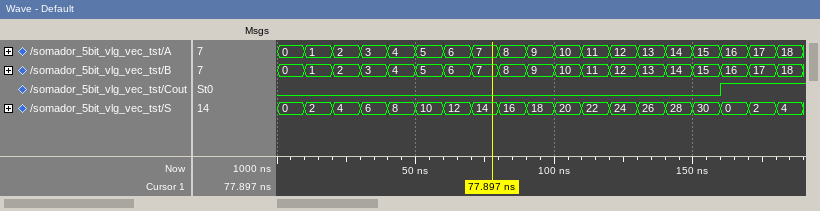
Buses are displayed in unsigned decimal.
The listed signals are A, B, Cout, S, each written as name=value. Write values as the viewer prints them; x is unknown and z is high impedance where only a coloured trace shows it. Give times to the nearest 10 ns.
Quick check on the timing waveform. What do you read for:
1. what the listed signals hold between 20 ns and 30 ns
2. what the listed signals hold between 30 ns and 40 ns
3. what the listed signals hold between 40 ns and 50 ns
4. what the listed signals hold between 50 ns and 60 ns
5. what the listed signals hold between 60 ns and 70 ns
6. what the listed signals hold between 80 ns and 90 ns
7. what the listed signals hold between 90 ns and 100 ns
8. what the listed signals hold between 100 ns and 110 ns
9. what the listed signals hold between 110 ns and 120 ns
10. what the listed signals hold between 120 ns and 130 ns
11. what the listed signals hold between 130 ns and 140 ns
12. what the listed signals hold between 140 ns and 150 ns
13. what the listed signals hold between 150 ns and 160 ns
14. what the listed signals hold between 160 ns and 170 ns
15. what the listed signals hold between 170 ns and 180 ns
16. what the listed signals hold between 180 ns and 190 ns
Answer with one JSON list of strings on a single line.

["A=2, B=2, Cout=0, S=4", "A=3, B=3, Cout=0, S=6", "A=4, B=4, Cout=0, S=8", "A=5, B=5, Cout=0, S=10", "A=6, B=6, Cout=0, S=12", "A=8, B=8, Cout=0, S=16", "A=9, B=9, Cout=0, S=18", "A=10, B=10, Cout=0, S=20", "A=11, B=11, Cout=0, S=22", "A=12, B=12, Cout=0, S=24", "A=13, B=13, Cout=0, S=26", "A=14, B=14, Cout=0, S=28", "A=15, B=15, Cout=0, S=30", "A=16, B=16, Cout=1, S=0", "A=17, B=17, Cout=1, S=2", "A=18, B=18, Cout=1, S=4"]
